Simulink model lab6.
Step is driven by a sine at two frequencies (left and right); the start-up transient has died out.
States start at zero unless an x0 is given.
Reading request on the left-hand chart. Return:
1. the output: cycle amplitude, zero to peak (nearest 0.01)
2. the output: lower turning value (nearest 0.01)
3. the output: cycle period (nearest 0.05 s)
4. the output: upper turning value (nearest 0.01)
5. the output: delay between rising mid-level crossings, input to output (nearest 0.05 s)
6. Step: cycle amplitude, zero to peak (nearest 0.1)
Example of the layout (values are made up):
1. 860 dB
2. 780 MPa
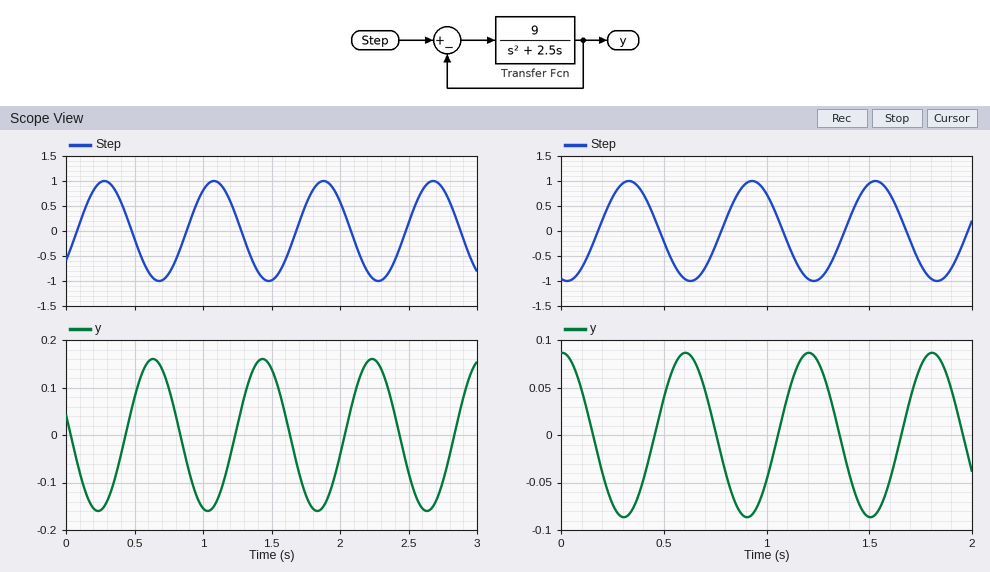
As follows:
1. 0.16
2. -0.16
3. 0.80 s
4. 0.16
5. 0.35 s
6. 1.0
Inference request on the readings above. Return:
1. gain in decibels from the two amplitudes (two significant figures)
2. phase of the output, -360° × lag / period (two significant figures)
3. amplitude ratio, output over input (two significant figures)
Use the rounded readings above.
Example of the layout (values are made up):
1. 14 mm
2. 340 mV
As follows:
1. -16 dB
2. -160°
3. 0.16
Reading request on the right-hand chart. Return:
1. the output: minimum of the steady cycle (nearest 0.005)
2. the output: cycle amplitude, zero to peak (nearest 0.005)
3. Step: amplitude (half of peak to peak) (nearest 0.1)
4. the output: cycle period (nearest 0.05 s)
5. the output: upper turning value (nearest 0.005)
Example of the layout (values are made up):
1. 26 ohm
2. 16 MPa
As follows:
1. -0.085
2. 0.085
3. 1.0
4. 0.60 s
5. 0.085
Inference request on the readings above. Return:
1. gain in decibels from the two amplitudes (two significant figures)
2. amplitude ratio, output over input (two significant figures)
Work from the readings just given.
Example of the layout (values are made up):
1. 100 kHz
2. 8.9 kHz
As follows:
1. -21 dB
2. 0.085
